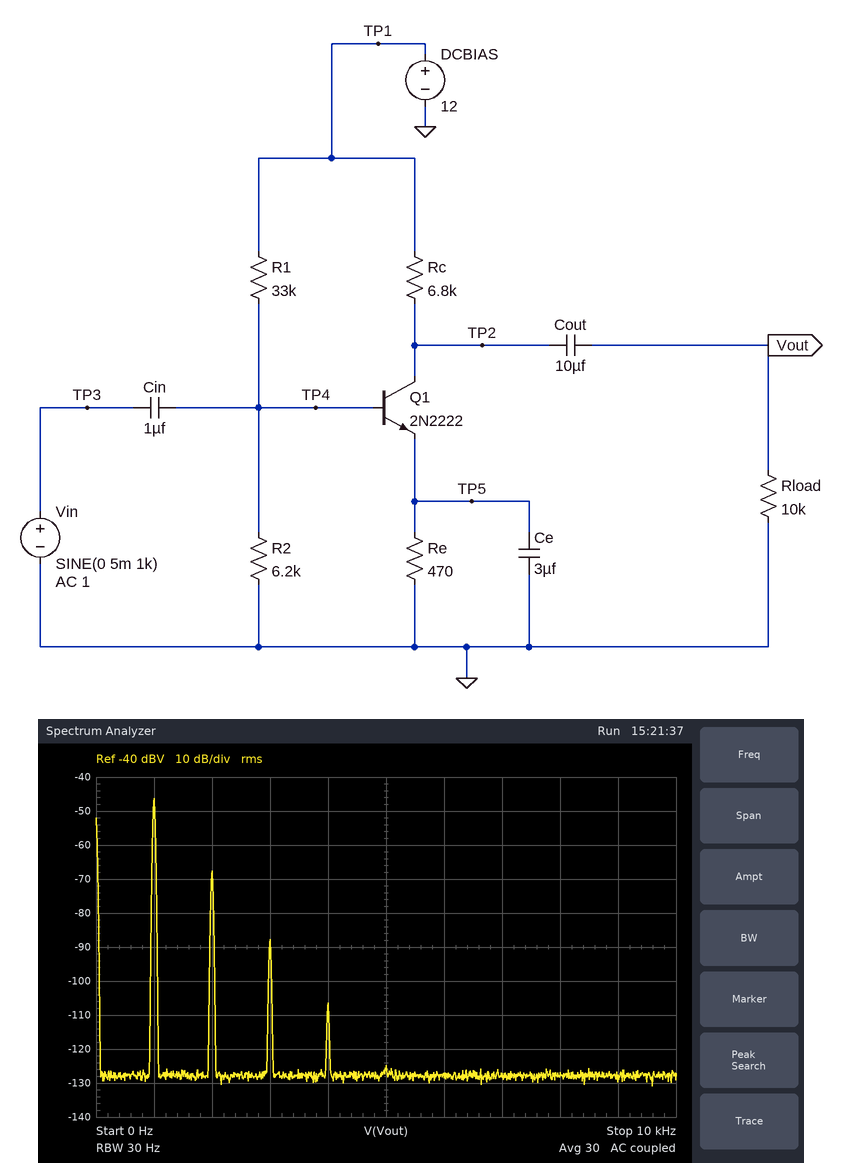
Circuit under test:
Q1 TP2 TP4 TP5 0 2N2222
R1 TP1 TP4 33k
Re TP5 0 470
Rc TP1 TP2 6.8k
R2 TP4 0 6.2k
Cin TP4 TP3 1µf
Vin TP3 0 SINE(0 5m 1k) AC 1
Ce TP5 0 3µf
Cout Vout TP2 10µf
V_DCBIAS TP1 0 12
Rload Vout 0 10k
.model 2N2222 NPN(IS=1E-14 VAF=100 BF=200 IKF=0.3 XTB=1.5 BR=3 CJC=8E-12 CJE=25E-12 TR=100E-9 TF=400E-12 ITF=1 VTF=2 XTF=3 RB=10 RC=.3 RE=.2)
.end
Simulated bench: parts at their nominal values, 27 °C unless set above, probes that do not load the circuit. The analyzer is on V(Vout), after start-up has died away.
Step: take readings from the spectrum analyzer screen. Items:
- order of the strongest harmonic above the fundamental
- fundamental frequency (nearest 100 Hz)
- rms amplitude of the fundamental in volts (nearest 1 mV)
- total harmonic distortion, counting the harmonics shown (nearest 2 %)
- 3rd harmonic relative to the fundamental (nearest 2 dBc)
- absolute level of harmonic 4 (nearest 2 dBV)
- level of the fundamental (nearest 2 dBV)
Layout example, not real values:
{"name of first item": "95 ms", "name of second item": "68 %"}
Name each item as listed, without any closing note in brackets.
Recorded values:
{"order of the strongest harmonic above the fundamental": "2", "fundamental frequency": "1.0 kHz", "rms amplitude of the fundamental in volts": "5 mV", "total harmonic distortion, counting the harmonics shown": "8 %", "3rd harmonic relative to the fundamental": "-42 dBc", "absolute level of harmonic 4": "-106 dBV", "level of the fundamental": "-46 dBV"}
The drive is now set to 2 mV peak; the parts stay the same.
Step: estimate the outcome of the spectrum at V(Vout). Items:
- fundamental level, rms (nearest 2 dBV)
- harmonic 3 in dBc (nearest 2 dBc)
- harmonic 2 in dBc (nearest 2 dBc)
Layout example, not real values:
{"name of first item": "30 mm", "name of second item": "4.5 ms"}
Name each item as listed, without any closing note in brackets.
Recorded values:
{"fundamental level, rms": "-54 dBV", "harmonic 3 in dBc": "-58 dBc", "harmonic 2 in dBc": "-30 dBc"}
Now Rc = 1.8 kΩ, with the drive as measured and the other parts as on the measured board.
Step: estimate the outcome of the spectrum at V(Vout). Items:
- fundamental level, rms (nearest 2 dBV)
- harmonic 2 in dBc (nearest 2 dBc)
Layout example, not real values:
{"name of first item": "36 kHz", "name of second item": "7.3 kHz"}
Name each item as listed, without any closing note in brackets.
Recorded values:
{"fundamental level, rms": "-20 dBV", "harmonic 2 in dBc": "-50 dBc"}
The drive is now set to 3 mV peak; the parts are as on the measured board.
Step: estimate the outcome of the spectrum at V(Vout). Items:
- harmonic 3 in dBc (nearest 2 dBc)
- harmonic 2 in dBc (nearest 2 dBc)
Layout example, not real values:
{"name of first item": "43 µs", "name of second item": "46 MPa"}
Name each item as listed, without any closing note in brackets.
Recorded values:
{"harmonic 3 in dBc": "-50 dBc", "harmonic 2 in dBc": "-26 dBc"}
